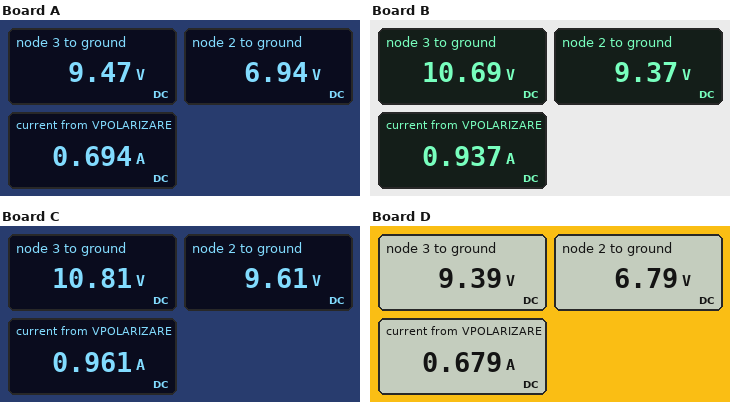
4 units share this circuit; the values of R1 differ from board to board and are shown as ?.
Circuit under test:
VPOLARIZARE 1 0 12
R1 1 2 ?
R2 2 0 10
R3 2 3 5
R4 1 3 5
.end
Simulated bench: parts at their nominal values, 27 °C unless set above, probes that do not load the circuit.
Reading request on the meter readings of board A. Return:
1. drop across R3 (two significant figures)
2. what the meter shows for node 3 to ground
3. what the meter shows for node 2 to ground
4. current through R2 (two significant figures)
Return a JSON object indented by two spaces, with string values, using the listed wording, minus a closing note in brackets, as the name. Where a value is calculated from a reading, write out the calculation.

{
  "drop across R3": "9.47 V - 6.94 V = 2.5 V",
  "what the meter shows for node 3 to ground": "9.47 V",
  "what the meter shows for node 2 to ground": "6.94 V",
  "current through R2": "(6.94 V) / 10 Ω = 690 mA"
}
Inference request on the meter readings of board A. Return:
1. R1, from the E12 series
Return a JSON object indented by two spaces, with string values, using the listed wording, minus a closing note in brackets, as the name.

{
  "R1, from the E12 series": "27 Ω"
}
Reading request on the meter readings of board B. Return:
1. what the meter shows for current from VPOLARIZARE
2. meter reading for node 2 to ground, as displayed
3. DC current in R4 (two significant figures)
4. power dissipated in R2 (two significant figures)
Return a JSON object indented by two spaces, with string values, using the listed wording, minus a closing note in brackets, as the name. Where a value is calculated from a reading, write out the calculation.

{
  "what the meter shows for current from VPOLARIZARE": "0.937 A",
  "meter reading for node 2 to ground, as displayed": "9.37 V",
  "DC current in R4": "(12 V - 10.69 V) / 5 Ω = 260 mA",
  "power dissipated in R2": "(9.37 V)^2 / 10 Ω = 8.8 W"
}
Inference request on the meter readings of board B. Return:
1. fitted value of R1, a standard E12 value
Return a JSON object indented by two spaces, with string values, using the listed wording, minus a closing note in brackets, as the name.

{
  "fitted value of R1, a standard E12 value": "3.9 Ω"
}
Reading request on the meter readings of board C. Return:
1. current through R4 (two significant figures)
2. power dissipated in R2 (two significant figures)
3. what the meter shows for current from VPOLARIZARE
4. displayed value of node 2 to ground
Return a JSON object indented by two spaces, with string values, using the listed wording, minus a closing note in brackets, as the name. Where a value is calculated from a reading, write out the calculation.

{
  "current through R4": "(12 V - 10.81 V) / 5 Ω = 240 mA",
  "power dissipated in R2": "(9.61 V)^2 / 10 Ω = 9.2 W",
  "what the meter shows for current from VPOLARIZARE": "0.961 A",
  "displayed value of node 2 to ground": "9.61 V"
}
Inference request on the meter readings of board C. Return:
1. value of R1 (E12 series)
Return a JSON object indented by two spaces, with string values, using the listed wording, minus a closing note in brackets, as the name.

{
  "value of R1": "3.3 Ω"
}
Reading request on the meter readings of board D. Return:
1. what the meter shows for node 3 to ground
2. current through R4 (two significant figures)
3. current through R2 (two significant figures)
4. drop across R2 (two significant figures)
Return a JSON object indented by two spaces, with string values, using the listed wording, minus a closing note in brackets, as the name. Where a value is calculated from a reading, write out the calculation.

{
  "what the meter shows for node 3 to ground": "9.39 V",
  "current through R4": "(12 V - 9.39 V) / 5 Ω = 520 mA",
  "current through R2": "(6.79 V) / 10 Ω = 680 mA",
  "drop across R2": "6.79 V = 6.8 V"
}
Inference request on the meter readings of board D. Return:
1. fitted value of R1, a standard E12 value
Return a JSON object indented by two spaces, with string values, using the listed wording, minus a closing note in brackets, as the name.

{
  "fitted value of R1, a standard E12 value": "33 Ω"
}
